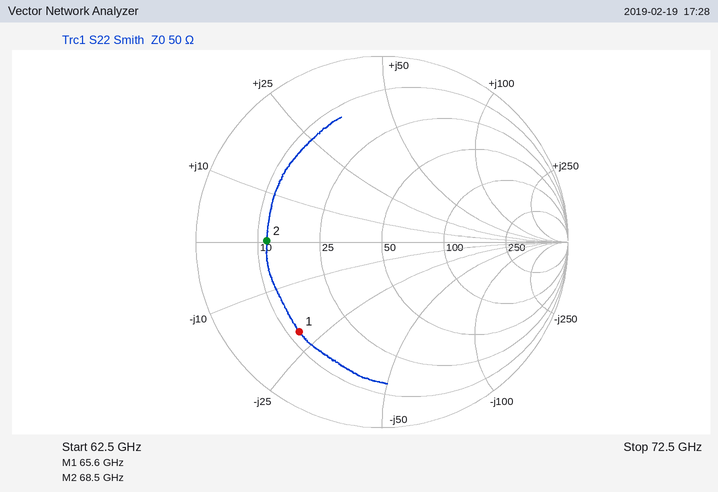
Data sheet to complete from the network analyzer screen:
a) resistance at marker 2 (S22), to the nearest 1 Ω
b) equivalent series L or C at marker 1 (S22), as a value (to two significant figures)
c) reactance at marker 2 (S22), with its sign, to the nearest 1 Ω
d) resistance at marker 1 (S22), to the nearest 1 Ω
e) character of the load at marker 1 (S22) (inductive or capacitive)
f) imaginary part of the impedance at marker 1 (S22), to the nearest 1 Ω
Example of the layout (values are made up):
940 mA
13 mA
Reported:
12 Ω
120 fF
0 Ω
12 Ω
capacitive
-21 Ω
